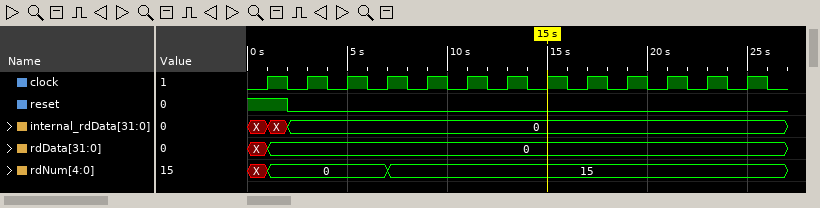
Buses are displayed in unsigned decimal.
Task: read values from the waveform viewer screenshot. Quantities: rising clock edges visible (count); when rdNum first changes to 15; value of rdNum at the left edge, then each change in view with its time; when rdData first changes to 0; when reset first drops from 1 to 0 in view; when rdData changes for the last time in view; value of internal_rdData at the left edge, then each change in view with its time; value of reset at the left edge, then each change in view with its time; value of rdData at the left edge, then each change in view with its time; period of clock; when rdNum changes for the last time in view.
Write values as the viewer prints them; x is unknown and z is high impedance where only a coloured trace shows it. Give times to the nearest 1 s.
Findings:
13
7 s
X, 0 at 1 s, 15 at 7 s
1 s
2 s
1 s
X, X at 1 s, 0 at 2 s
1, 0 at 2 s
X, 0 at 1 s
2 s
7 s
